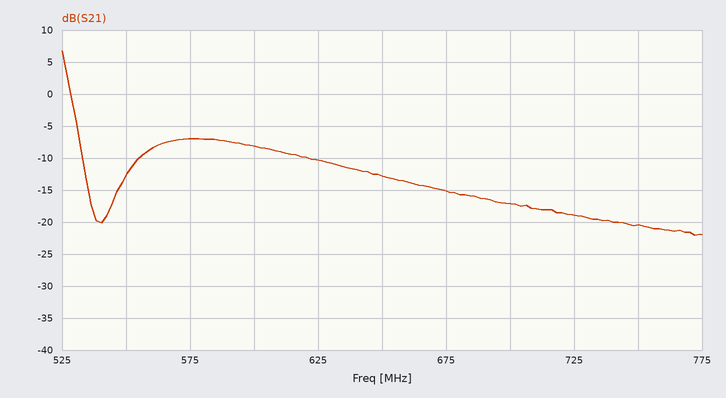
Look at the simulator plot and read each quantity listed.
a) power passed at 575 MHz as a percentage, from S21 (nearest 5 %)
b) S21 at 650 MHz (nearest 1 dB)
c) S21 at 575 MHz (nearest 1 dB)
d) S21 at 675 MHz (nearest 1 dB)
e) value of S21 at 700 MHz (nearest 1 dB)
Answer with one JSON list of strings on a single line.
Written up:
["20 %", "-13 dB", "-7 dB", "-15 dB", "-17 dB"]
